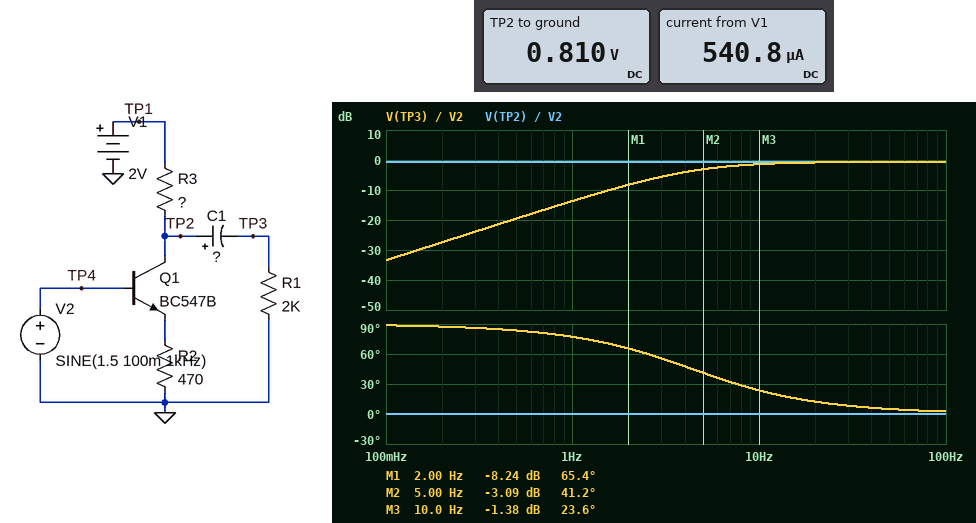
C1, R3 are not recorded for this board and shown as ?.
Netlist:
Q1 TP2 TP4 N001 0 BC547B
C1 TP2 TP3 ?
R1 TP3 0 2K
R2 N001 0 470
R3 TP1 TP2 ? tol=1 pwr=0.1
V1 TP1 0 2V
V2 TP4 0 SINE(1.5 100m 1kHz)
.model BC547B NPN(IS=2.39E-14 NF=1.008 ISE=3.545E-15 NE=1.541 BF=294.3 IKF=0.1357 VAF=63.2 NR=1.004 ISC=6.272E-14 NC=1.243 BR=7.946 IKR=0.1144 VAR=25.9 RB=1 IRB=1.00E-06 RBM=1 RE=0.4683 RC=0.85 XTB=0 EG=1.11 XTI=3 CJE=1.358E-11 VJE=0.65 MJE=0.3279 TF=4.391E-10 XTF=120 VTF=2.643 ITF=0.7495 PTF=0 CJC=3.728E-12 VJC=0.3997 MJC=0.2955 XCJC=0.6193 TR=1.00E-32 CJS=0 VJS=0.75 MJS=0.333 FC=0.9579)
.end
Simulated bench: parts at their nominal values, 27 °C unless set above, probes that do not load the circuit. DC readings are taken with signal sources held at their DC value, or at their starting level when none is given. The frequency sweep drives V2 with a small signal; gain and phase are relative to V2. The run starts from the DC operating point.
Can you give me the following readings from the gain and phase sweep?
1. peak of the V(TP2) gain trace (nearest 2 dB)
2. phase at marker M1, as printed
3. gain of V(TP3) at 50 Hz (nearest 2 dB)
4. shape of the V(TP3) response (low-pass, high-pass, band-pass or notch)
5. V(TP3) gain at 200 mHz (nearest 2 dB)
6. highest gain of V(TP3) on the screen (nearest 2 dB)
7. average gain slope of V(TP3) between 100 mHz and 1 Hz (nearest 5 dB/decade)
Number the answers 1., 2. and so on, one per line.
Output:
1. 0 dB
2. 65.4 deg
3. 0 dB
4. high-pass
5. -28 dB
6. 0 dB
7. 20 dB/decade
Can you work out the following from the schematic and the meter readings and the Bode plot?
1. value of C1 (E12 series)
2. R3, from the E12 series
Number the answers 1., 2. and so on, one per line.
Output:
1. 18 µF
2. 2.2 kΩ
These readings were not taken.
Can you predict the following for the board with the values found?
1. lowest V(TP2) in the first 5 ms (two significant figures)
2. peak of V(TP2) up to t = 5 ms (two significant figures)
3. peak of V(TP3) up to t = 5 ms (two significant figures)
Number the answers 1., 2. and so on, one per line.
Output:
1. 720 mV
2. 900 mV
3. 93 mV
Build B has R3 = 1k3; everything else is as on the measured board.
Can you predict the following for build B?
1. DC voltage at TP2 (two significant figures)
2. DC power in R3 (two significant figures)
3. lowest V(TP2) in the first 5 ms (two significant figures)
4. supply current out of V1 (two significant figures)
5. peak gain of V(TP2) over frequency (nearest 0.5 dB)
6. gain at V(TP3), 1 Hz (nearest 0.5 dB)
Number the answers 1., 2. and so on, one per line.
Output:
1. 820 mV
2. 1.1 mW
3. 730 mV
4. 910 µA
5. -1.0 dB
6. -14.0 dB
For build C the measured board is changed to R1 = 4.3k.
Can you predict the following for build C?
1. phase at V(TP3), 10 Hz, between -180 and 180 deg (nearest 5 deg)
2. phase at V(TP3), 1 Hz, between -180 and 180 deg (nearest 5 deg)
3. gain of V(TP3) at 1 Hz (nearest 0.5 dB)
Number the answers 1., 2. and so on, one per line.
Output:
1. 10 deg
2. 65 deg
3. -7.5 dB
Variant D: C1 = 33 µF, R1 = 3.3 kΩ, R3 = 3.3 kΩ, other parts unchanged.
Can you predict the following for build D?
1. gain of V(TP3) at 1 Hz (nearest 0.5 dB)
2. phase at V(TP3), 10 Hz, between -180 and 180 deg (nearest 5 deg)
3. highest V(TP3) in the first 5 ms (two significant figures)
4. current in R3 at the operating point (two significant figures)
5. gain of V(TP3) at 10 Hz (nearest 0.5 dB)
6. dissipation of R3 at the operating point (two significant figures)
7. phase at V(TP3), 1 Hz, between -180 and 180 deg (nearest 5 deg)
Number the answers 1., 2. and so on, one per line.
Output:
1. -5.5 dB
2. 10 deg
3. 95 mV
4. 360 µA
5. -0.5 dB
6. 430 µW
7. 55 deg
